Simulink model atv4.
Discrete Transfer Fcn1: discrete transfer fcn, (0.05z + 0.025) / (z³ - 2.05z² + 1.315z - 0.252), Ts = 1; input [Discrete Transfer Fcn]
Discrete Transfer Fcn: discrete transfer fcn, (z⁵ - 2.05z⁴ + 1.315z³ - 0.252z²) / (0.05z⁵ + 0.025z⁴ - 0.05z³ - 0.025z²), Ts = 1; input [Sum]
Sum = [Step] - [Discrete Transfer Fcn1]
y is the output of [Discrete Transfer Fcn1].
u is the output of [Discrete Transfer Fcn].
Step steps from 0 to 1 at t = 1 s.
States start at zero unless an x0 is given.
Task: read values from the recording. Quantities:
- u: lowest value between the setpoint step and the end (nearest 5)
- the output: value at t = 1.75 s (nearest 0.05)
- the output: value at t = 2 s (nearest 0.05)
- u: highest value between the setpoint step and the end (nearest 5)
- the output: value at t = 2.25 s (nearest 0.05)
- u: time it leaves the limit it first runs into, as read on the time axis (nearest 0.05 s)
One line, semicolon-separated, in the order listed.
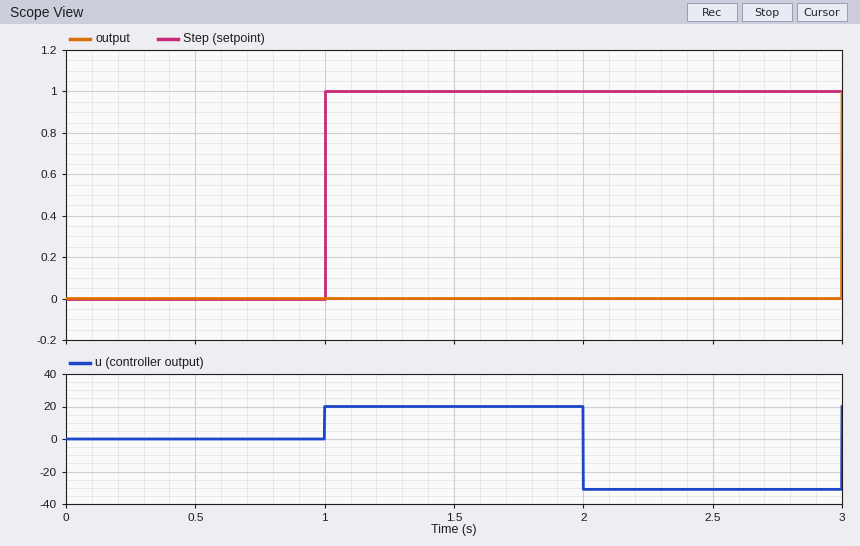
-30; 0.00; 0.00; 20; 0.00; 2.00 s
